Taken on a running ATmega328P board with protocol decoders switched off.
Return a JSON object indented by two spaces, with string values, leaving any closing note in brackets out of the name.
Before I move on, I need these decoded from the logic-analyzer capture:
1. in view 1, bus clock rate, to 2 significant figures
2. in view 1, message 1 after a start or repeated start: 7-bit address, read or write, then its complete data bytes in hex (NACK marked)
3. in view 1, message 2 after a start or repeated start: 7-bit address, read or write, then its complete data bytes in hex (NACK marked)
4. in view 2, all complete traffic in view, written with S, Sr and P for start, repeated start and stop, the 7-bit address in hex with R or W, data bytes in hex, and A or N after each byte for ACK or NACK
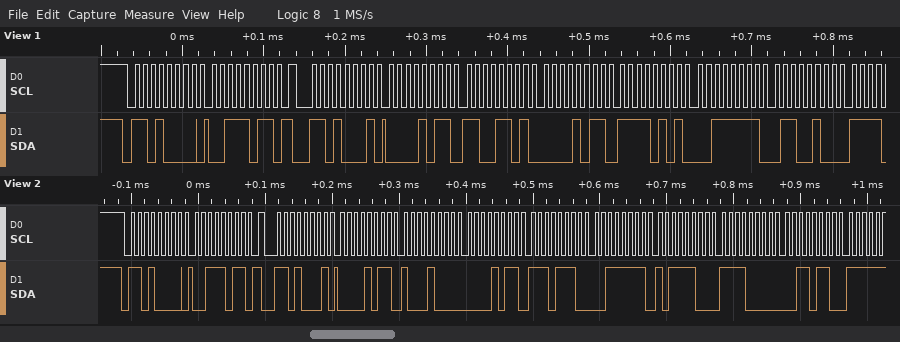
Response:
{
  "in view 1, bus clock rate, to 2 significant figures": "100 kHz",
  "in view 1, message 1 after a start or repeated start: 7-bit address, read or write, then its complete data bytes in hex": "0x68 write: 3B",
  "in view 1, message 2 after a start or repeated start: 7-bit address, read or write, then its complete data bytes in hex": "0x68 read: 0B CD 0B F5 3F 64",
  "in view 2, all complete traffic in view, written with S, Sr and P for start, repeated start and stop, the 7-bit address in hex with R or W, data bytes in hex, and A or N after each byte for ACK or NACK": "S 68W A 3B A Sr 68R A 0B A 88 A 0B A EE A 3F A BC A F0 A 36 A"
}
